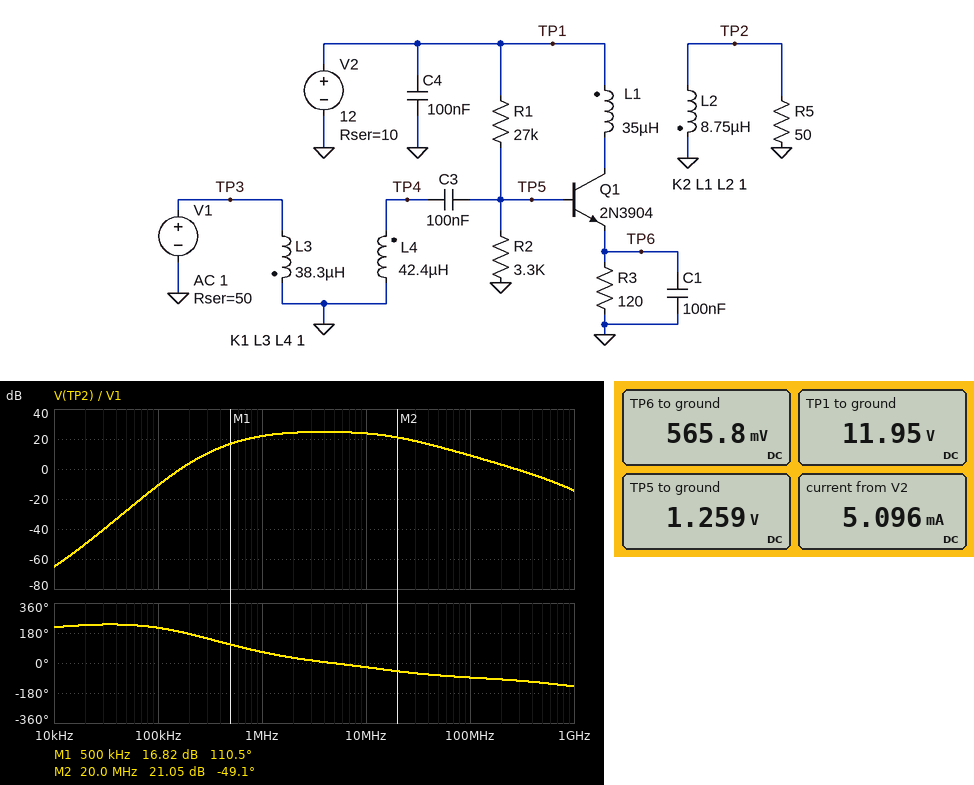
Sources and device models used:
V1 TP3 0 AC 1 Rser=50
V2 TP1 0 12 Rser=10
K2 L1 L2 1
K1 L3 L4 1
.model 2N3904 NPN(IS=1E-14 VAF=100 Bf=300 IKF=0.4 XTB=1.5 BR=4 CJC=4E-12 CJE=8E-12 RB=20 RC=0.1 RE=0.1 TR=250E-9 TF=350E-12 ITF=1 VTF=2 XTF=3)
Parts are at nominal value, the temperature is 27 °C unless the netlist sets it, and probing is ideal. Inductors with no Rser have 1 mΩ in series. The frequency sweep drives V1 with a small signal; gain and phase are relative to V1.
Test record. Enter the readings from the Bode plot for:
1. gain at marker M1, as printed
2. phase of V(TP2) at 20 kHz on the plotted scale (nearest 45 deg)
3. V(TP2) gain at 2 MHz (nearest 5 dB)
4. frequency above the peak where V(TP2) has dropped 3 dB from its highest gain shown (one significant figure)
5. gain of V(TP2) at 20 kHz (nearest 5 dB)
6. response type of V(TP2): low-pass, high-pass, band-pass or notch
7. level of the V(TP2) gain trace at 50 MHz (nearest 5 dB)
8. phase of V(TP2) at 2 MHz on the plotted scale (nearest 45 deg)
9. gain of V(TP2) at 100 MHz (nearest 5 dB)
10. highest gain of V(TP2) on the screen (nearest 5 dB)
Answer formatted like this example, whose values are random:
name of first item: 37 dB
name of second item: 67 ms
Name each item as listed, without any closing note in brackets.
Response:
gain at marker M1, as printed: 16.82 dB
phase of V(TP2) at 20 kHz on the plotted scale: 225 deg
V(TP2) gain at 2 MHz: 25 dB
frequency above the peak where V(TP2) has dropped 3 dB from its highest gain shown: 20 MHz
gain of V(TP2) at 20 kHz: -50 dB
response type of V(TP2): low-pass, high-pass, band-pass or notch: band-pass
level of the V(TP2) gain trace at 50 MHz: 15 dB
phase of V(TP2) at 2 MHz on the plotted scale: 45 deg
gain of V(TP2) at 100 MHz: 10 dB
highest gain of V(TP2) on the screen: 25 dB
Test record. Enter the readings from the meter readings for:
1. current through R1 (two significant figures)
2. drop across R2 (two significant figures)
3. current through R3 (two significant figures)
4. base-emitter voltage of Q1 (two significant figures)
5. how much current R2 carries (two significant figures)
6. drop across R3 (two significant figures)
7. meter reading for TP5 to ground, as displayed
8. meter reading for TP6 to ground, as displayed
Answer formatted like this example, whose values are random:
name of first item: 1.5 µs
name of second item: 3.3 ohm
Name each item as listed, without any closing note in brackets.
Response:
current through R1: 400 µA
drop across R2: 1.3 V
current through R3: 4.7 mA
base-emitter voltage of Q1: 690 mV
how much current R2 carries: 380 µA
drop across R3: 570 mV
meter reading for TP5 to ground, as displayed: 1.259 V
meter reading for TP6 to ground, as displayed: 565.8 mV
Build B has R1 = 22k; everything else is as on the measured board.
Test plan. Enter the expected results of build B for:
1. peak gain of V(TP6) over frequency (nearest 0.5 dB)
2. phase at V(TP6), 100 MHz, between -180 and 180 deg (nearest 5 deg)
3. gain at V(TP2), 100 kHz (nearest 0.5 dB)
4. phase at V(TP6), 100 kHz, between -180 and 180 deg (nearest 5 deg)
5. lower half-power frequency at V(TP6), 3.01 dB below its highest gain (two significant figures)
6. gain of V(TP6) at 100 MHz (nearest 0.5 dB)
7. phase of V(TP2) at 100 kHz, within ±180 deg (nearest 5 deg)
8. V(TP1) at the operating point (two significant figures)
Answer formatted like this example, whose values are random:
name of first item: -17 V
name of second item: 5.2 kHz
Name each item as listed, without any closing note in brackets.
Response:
peak gain of V(TP6) over frequency: -3.5 dB
phase at V(TP6), 100 MHz, between -180 and 180 deg: 25 deg
gain at V(TP2), 100 kHz: -10.5 dB
phase at V(TP6), 100 kHz, between -180 and 180 deg: -130 deg
lower half-power frequency at V(TP6), 3.01 dB below its highest gain: 110 kHz
gain of V(TP6) at 100 MHz: -66.0 dB
phase of V(TP2) at 100 kHz, within ±180 deg: -145 deg
V(TP1) at the operating point: 12 V
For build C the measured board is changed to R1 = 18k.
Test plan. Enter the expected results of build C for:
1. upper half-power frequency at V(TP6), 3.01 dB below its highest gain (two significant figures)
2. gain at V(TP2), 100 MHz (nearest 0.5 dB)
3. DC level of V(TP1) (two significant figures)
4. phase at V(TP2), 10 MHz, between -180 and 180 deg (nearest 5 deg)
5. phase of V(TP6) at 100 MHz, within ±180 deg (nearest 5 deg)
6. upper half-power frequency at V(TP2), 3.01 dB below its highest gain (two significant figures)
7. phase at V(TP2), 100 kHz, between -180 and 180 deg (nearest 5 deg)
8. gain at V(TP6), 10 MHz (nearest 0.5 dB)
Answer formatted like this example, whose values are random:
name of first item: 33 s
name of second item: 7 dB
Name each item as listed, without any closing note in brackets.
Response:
upper half-power frequency at V(TP6), 3.01 dB below its highest gain: 850 kHz
gain at V(TP2), 100 MHz: 9.5 dB
DC level of V(TP1): 12 V
phase at V(TP2), 10 MHz, between -180 and 180 deg: -40 deg
phase of V(TP6) at 100 MHz, within ±180 deg: 25 deg
upper half-power frequency at V(TP2), 3.01 dB below its highest gain: 11 MHz
phase at V(TP2), 100 kHz, between -180 and 180 deg: -140 deg
gain at V(TP6), 10 MHz: -29.0 dB
